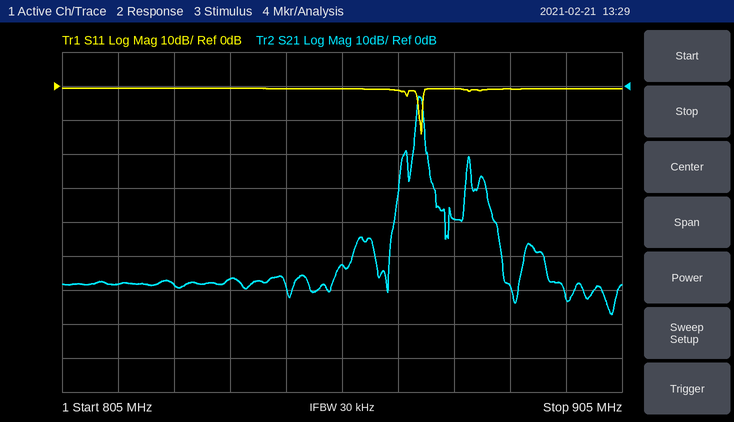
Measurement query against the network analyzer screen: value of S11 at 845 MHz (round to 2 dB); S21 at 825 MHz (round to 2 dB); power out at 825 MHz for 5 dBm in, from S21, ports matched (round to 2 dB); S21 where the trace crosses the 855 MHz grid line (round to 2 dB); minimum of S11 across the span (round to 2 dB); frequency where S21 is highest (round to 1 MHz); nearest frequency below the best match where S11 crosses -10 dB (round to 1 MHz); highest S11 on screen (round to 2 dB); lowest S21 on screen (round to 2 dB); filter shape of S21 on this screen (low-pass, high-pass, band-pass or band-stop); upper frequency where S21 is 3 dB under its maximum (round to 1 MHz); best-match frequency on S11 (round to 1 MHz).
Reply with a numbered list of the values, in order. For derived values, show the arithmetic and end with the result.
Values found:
1. 0 dB
2. -58 dB
3. 5 dBm + (-58 dB) = -54 dBm
4. -52 dB
5. -14 dB
6. 869 MHz
7. 869 MHz
8. 0 dB
9. -68 dB
10. band-pass
11. 869 MHz
12. 869 MHz
